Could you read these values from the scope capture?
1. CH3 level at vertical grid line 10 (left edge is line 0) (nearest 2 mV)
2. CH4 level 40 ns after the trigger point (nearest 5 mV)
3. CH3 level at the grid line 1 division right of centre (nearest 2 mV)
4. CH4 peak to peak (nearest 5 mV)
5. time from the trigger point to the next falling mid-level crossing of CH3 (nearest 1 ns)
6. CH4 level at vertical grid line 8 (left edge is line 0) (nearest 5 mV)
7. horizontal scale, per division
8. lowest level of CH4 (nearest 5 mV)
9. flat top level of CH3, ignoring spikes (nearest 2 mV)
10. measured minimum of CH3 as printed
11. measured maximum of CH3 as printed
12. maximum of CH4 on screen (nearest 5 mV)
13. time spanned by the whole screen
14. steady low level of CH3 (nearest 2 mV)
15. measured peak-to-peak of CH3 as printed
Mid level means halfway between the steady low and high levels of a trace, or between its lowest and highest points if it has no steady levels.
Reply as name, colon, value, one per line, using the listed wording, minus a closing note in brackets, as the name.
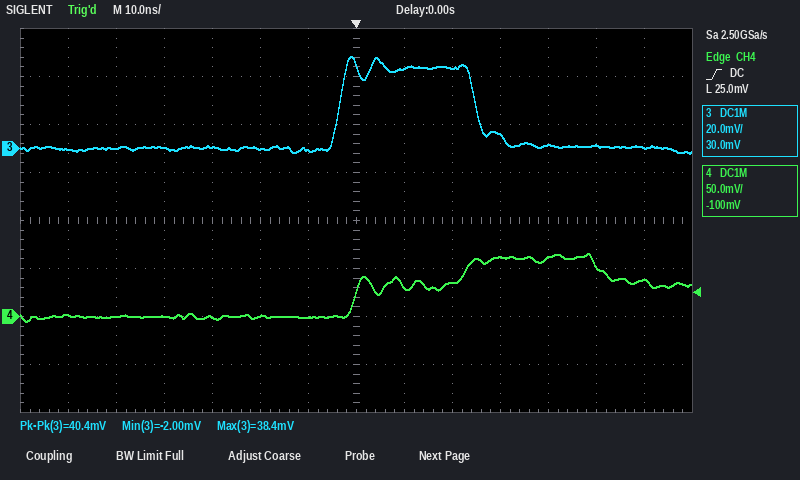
CH3 level at vertical grid line 10 (left edge is line 0): 6 mV
CH4 level 40 ns after the trigger point: 60 mV
CH3 level at the grid line 1 division right of centre: 34 mV
CH4 peak to peak: 70 mV
time from the trigger point to the next falling mid-level crossing of CH3: 25 ns
CH4 level at vertical grid line 8 (left edge is line 0): 30 mV
horizontal scale, per division: 10 ns
lowest level of CH4: -5 mV
flat top level of CH3, ignoring spikes: 34 mV
measured minimum of CH3 as printed: -2.00 mV
measured maximum of CH3 as printed: 38.4 mV
maximum of CH4 on screen: 65 mV
time spanned by the whole screen: 140 ns
steady low level of CH3: 0 mV
measured peak-to-peak of CH3 as printed: 40.4 mV
